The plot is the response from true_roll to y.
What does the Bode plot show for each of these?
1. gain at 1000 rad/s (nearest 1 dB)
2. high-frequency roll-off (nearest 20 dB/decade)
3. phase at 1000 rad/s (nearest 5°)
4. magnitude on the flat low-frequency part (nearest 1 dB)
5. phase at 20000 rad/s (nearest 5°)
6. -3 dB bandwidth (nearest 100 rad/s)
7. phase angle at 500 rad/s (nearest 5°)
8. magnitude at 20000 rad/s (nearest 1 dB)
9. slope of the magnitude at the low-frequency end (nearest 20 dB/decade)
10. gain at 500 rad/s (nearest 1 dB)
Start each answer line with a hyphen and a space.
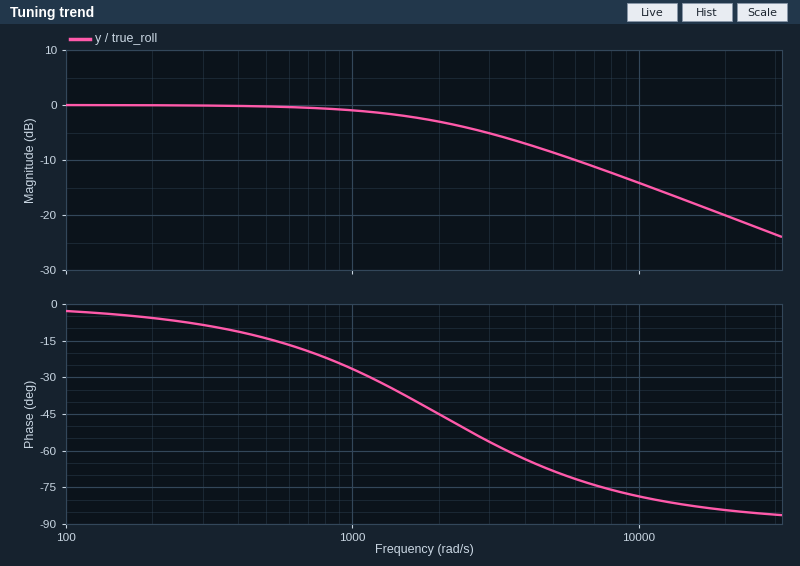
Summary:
- -1 dB
- -20 dB/decade
- -25°
- 0 dB
- -85°
- 2000 rad/s
- -15°
- -20 dB
- 0 dB/decade
- 0 dB
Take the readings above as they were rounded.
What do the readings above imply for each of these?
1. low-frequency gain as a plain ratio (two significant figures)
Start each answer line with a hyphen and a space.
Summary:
- 1.0
